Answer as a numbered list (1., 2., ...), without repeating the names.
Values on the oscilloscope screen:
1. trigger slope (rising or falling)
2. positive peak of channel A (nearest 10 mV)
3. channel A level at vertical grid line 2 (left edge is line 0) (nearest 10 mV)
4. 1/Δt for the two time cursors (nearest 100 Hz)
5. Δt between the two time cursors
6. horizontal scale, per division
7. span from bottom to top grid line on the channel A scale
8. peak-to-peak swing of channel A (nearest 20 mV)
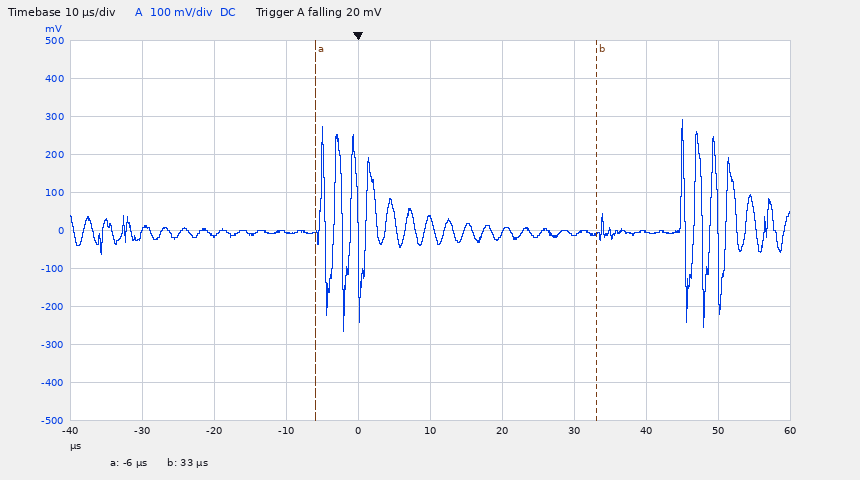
1. falling
2. 290 mV
3. -10 mV
4. 25.6 kHz
5. 39 µs
6. 10 µs
7. 1 V
8. 560 mV
